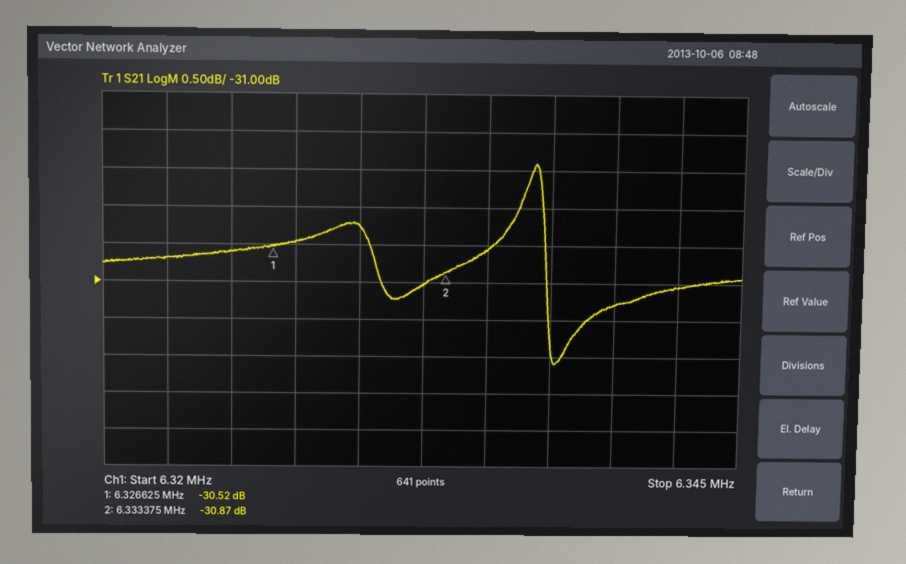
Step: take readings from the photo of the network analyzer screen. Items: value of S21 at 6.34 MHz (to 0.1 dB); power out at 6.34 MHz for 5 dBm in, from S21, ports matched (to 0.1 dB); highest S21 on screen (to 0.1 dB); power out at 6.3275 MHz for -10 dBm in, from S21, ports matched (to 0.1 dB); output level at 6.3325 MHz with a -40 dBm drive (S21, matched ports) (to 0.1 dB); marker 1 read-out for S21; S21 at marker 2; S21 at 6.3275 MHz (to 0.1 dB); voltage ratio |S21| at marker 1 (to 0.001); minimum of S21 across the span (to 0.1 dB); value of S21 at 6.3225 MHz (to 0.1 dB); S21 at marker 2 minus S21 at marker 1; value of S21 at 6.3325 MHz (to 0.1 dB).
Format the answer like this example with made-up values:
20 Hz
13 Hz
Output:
-31.3 dB
-26.3 dBm
-29.4 dB
-40.5 dBm
-71.0 dBm
-30.52 dB
-30.87 dB
-30.5 dB
0.030
-32.1 dB
-30.7 dB
-0.35 dB
-31.0 dB
